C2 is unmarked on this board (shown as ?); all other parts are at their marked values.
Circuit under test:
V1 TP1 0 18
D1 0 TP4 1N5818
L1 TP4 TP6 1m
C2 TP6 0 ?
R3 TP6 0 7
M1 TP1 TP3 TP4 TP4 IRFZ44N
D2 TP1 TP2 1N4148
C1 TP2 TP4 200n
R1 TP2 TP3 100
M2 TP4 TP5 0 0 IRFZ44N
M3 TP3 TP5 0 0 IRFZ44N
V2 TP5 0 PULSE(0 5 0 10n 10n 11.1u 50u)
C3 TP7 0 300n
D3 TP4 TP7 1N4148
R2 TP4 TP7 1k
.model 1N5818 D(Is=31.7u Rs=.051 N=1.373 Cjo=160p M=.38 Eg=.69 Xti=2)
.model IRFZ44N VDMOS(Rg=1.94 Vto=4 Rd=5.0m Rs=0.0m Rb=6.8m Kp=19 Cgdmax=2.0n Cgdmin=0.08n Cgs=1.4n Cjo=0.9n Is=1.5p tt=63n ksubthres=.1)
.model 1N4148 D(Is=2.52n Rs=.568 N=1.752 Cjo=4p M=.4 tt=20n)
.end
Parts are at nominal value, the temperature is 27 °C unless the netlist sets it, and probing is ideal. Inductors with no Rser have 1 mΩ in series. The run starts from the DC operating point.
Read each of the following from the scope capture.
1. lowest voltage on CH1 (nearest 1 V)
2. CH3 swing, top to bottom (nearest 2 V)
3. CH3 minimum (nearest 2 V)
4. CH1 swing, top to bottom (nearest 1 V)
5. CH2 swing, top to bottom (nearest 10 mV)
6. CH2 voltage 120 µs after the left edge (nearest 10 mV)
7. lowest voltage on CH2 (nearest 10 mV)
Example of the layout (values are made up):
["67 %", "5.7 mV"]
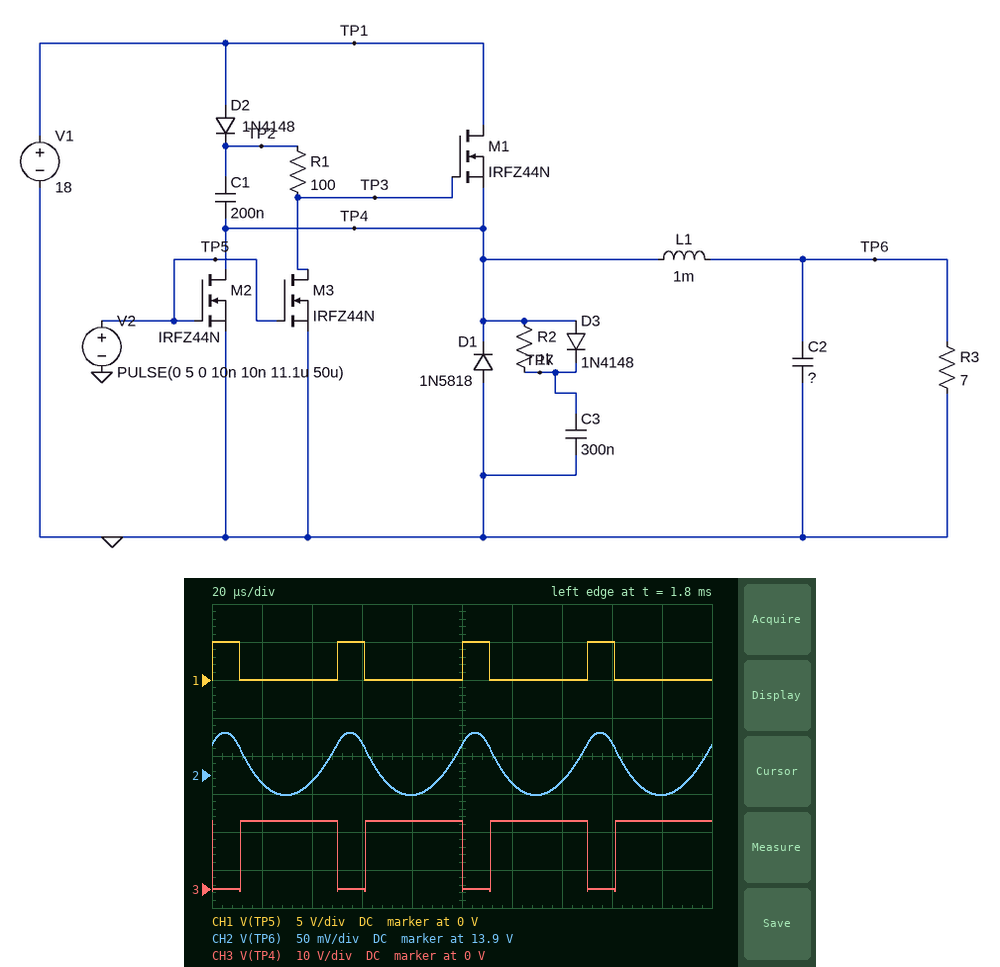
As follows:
["0 V", "18 V", "0 V", "5 V", "80 mV", "13.89 V", "13.87 V"]
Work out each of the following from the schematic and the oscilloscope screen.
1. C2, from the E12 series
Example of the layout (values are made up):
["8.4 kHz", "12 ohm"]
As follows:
["12 µF"]
